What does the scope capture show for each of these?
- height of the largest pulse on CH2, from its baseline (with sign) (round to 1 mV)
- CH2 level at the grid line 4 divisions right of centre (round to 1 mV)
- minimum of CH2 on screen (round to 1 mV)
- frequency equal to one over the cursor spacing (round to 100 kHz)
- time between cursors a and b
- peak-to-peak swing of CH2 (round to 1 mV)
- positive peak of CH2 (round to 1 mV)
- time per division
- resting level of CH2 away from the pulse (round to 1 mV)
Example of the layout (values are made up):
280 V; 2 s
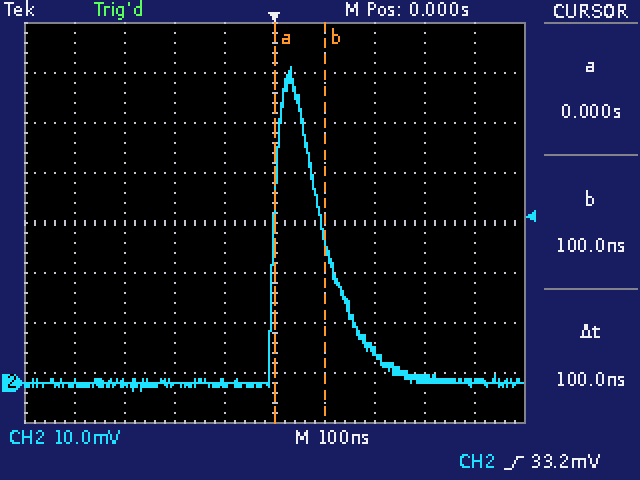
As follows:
+63 mV; 0 mV; -2 mV; 10.0 MHz; 100 ns; 65 mV; 63 mV; 100 ns; 0 mV
